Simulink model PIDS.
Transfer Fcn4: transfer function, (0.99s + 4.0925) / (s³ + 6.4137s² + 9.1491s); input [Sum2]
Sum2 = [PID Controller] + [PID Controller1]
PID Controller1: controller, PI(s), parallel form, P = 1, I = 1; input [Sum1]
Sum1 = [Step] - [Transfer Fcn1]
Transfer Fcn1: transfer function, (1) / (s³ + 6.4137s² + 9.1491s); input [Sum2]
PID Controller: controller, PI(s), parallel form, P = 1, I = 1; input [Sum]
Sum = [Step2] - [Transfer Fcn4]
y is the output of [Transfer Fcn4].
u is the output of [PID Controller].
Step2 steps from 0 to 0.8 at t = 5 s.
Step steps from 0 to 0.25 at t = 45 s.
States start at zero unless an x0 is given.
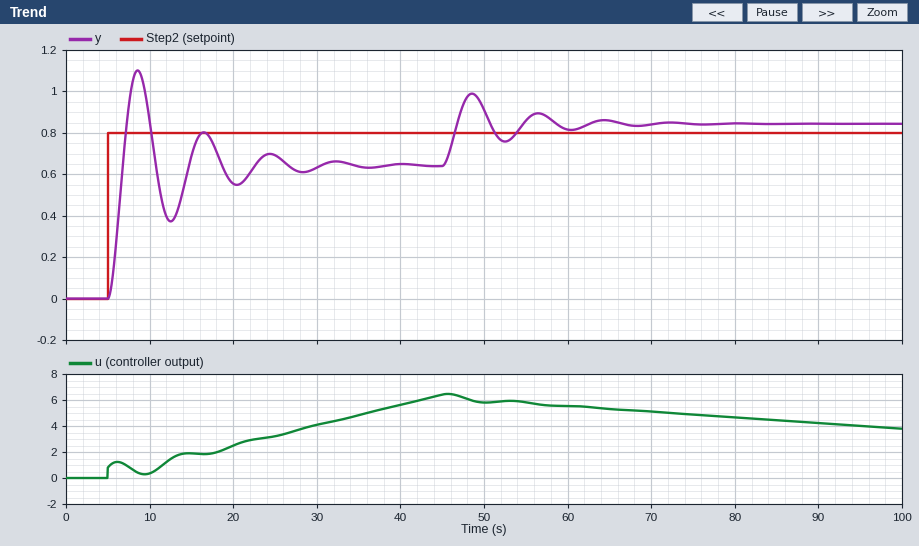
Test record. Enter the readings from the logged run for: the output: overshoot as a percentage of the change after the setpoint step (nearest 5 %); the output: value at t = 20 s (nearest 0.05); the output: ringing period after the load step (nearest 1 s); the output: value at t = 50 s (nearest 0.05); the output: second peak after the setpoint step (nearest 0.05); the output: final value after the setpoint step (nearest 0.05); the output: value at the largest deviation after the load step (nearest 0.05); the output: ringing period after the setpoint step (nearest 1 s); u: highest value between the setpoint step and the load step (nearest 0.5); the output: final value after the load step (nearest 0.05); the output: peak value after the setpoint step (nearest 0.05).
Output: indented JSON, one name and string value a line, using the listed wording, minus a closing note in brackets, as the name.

{
  "the output: overshoot as a percentage of the change after the setpoint step": "70 %",
  "the output: value at t = 20 s": "0.55",
  "the output: ringing period after the load step": "8 s",
  "the output: value at t = 50 s": "0.90",
  "the output: second peak after the setpoint step": "0.80",
  "the output: final value after the setpoint step": "0.65",
  "the output: value at the largest deviation after the load step": "1.00",
  "the output: ringing period after the setpoint step": "8 s",
  "u: highest value between the setpoint step and the load step": "6.5",
  "the output: final value after the load step": "0.85",
  "the output: peak value after the setpoint step": "1.10"
}
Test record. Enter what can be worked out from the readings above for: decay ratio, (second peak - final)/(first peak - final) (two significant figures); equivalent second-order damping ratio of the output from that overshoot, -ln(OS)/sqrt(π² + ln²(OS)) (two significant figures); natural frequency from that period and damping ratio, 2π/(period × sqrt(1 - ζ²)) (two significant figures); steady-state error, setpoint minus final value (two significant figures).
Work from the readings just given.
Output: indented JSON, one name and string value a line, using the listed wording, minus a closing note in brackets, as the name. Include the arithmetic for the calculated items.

{
  "decay ratio, (second peak - final)/(first peak - final)": "(0.8 - 0.65) / (1.1 - 0.65) = 0.33",
  "equivalent second-order damping ratio of the output from that overshoot, -ln(OS)/sqrt(π² + ln²(OS))": "ln(0.7) = -0.357; 0.357 / sqrt(9.870 + 0.127) = 0.11",
  "natural frequency from that period and damping ratio, 2π/(period × sqrt(1 - ζ²))": "2π / (8 × sqrt(1 - 0.11²)) = 0.79 rad/s",
  "steady-state error, setpoint minus final value": "0.8 - 0.65 = 0.15"
}
